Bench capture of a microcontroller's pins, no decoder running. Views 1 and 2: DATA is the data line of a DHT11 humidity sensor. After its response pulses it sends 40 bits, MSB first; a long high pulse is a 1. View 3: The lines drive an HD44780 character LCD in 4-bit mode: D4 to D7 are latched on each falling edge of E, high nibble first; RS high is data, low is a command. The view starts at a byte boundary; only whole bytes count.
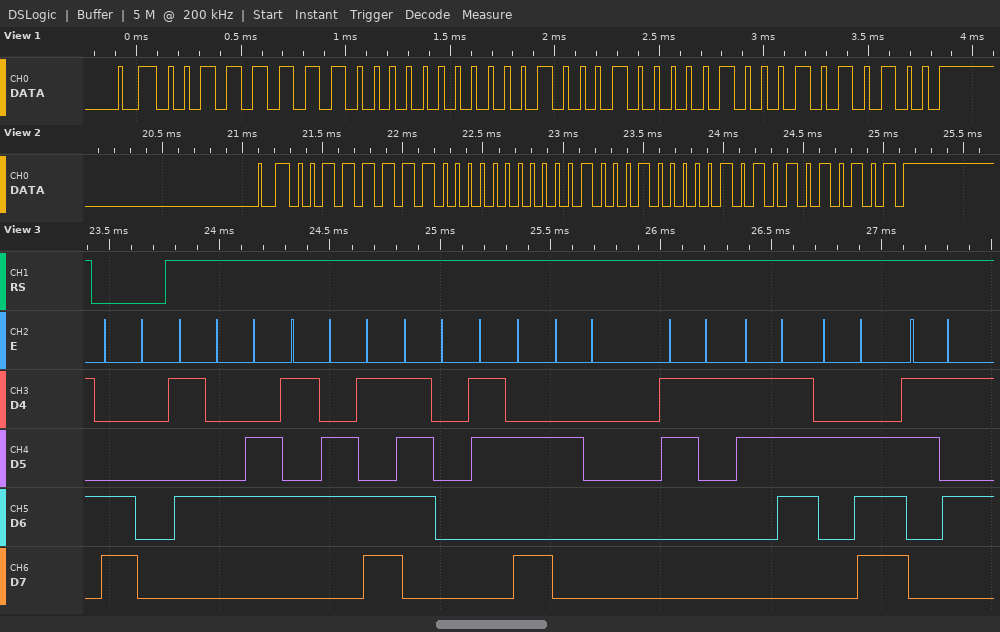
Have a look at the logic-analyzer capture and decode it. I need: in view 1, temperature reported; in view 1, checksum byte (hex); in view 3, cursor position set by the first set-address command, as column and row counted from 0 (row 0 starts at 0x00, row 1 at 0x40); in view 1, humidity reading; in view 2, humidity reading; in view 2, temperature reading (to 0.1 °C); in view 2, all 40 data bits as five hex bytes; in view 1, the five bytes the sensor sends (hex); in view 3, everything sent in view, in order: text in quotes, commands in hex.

17.4 °C
0x54
column 0, row 1
63 %
63 %
17.5 °C
3F 00 11 05 55
3F 00 11 04 54
0xC0 "Temp: 17.5"
